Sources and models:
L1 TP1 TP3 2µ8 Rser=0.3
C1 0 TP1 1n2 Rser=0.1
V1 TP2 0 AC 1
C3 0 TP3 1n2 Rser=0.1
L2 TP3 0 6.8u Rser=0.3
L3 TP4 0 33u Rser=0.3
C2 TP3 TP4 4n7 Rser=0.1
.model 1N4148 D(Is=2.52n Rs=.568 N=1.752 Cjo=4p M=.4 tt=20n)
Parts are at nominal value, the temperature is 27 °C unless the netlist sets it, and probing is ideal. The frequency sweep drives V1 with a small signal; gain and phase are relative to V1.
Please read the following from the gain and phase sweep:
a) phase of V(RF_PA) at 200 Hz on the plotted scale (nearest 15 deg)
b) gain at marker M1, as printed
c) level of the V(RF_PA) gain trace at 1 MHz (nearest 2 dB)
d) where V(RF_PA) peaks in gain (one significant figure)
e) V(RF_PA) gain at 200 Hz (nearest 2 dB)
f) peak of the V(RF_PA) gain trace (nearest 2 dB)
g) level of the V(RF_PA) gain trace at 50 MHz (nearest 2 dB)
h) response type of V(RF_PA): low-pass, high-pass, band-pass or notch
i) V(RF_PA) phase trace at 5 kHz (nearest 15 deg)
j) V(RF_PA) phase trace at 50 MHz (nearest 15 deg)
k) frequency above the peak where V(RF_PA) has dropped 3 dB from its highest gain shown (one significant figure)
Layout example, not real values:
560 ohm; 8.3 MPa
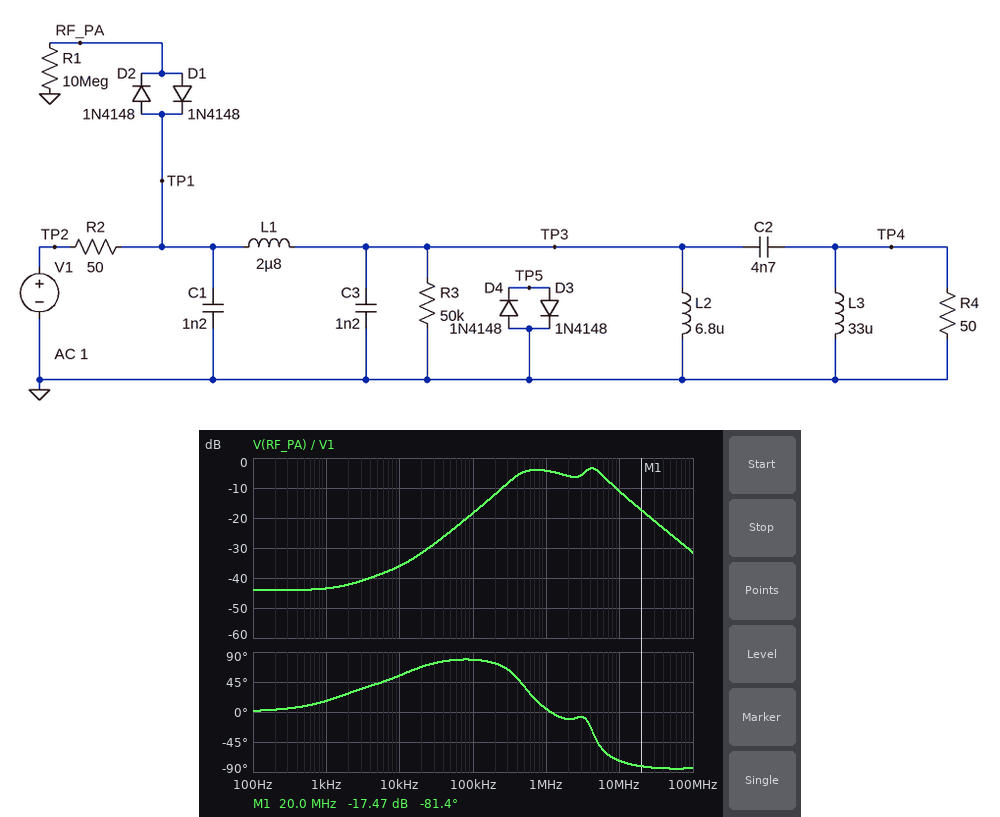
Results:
0 deg; -17.47 dB; -4 dB; 4 MHz; -44 dB; -4 dB; -26 dB; band-pass; 45 deg; -90 deg; 6 MHz
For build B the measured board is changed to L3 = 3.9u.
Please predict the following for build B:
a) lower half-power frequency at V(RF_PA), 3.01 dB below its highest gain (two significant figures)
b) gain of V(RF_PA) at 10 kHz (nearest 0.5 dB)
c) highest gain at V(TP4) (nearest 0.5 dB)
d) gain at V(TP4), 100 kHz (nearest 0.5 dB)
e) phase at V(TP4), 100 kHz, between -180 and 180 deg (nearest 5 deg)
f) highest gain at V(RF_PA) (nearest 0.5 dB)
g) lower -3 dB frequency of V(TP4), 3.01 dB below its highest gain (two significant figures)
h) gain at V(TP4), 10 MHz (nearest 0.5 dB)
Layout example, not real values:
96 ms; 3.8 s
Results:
440 kHz; -36.0 dB; -6.5 dB; -64.0 dB; -110 deg; -1.0 dB; 660 kHz; -32.5 dB
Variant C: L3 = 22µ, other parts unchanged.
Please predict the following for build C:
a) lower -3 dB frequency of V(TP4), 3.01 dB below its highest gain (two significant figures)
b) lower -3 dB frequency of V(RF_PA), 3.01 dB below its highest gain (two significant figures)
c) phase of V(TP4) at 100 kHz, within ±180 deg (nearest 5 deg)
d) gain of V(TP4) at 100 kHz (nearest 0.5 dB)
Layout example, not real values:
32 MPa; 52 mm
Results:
500 kHz; 360 kHz; -120 deg; -49.0 dB
